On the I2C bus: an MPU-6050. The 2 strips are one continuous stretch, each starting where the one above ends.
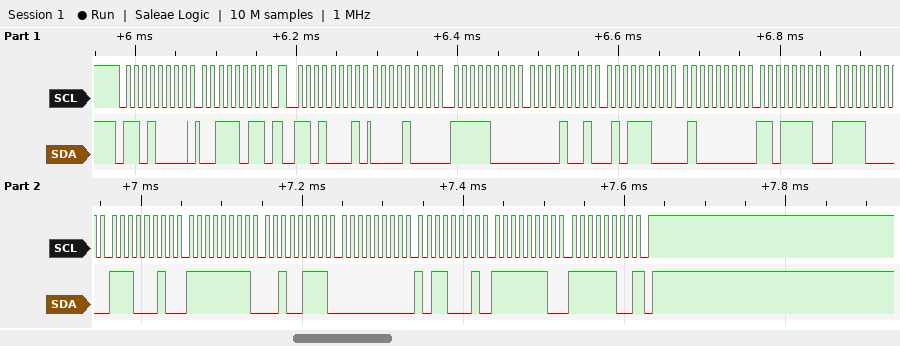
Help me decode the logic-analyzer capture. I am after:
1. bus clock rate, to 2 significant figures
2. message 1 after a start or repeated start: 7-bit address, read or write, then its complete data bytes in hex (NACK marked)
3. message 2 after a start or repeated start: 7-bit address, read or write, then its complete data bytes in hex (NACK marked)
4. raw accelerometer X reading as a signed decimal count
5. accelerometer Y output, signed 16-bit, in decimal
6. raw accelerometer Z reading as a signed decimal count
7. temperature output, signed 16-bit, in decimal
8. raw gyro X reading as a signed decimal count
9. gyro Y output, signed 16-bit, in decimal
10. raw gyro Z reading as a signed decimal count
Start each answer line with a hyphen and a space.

- 100 kHz
- 0x68 write: 3B
- 0x68 read: 08 F8 09 5C 40 DE F0 E2 FF 27 00 B1 FE FC NACK
- 2296
- 2396
- 16606
- -3870
- -217
- 177
- -260
